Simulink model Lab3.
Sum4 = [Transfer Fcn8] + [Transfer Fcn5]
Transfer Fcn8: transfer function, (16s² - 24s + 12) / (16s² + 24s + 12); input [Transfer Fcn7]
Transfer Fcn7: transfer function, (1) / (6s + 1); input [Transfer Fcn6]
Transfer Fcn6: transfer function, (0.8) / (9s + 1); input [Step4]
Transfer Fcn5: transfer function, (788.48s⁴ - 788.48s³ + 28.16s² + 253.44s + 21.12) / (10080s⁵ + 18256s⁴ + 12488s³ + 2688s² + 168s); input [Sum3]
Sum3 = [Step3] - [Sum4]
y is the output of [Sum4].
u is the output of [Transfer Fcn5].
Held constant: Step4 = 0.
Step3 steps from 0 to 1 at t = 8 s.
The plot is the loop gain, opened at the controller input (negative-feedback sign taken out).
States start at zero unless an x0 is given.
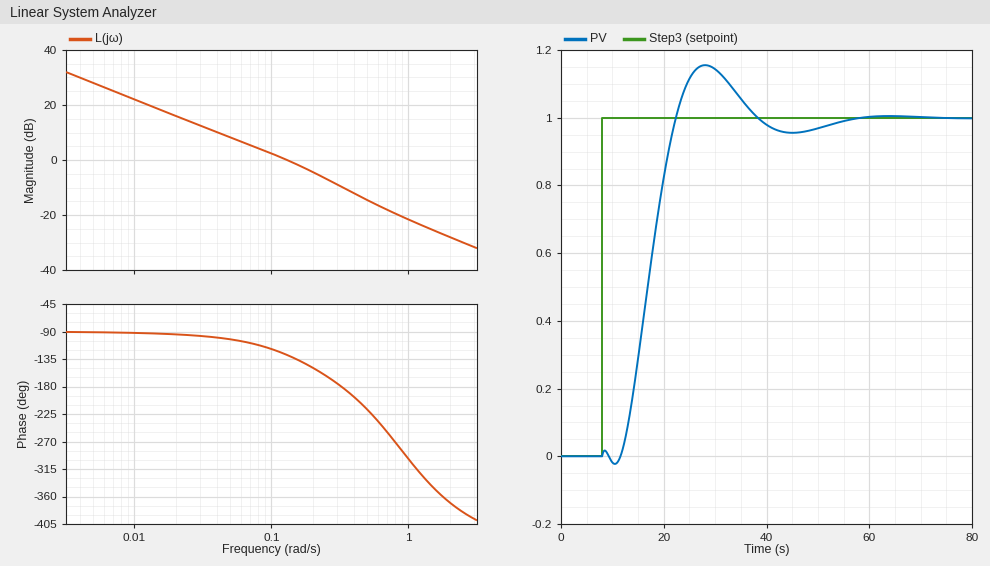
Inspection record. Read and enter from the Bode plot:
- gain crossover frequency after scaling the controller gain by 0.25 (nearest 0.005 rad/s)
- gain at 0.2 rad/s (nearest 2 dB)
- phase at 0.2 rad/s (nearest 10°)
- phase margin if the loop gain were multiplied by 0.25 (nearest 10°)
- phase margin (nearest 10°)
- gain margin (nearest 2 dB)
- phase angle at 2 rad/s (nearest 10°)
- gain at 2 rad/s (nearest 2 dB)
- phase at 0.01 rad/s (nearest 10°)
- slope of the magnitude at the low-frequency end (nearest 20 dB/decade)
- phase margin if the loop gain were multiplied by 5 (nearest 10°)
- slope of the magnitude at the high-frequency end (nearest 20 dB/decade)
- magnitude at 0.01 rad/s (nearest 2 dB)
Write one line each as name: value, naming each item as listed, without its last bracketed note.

gain crossover frequency after scaling the controller gain by 0.25: 0.030 rad/s
gain at 0.2 rad/s: -4 dB
phase at 0.2 rad/s: -150°
phase margin if the loop gain were multiplied by 0.25: 80°
phase margin: 50°
gain margin: 10 dB
phase angle at 2 rad/s: -370°
gain at 2 rad/s: -28 dB
phase at 0.01 rad/s: -90°
slope of the magnitude at the low-frequency end: -20 dB/decade
phase margin if the loop gain were multiplied by 5: -30°
slope of the magnitude at the high-frequency end: -20 dB/decade
magnitude at 0.01 rad/s: 22 dB
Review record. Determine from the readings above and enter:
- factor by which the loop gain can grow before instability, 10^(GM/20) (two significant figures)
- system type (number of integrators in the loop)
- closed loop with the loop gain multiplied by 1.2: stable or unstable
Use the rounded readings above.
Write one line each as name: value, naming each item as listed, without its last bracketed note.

factor by which the loop gain can grow before instability, 10^(GM/20): 3.2
system type: 1
closed loop with the loop gain multiplied by 1.2: stable or unstable: stable
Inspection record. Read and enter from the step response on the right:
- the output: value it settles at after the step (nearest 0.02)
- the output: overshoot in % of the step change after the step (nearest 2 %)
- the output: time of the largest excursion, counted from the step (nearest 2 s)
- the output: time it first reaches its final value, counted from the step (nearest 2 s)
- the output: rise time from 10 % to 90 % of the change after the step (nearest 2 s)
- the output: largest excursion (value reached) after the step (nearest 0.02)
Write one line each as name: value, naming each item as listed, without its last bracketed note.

the output: value it settles at after the step: 1.00
the output: overshoot in % of the step change after the step: 16 %
the output: time of the largest excursion, counted from the step: 20 s
the output: time it first reaches its final value, counted from the step: 14 s
the output: rise time from 10 % to 90 % of the change after the step: 8 s
the output: largest excursion (value reached) after the step: 1.16
